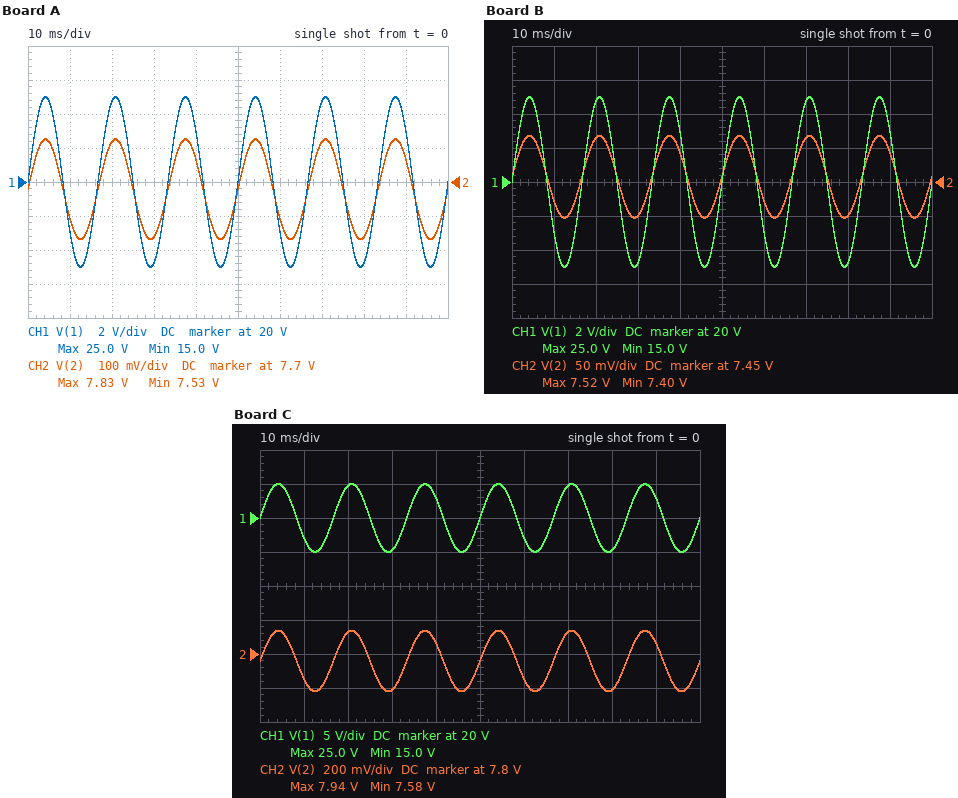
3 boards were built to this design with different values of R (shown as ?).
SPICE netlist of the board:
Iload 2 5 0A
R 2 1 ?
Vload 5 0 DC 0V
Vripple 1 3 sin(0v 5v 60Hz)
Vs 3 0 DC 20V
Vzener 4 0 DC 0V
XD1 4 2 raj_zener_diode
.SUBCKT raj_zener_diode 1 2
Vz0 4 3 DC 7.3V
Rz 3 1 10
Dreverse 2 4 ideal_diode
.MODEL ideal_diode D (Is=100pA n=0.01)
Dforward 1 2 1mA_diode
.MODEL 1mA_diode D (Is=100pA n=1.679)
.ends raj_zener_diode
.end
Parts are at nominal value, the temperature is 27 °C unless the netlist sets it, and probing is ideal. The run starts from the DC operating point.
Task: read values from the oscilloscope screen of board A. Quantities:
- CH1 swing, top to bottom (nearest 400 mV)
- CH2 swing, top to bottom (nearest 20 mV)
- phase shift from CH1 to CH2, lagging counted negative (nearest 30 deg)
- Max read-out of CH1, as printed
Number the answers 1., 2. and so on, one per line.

1. 10.0 V
2. 300 mV
3. 0 deg
4. 25.0 V
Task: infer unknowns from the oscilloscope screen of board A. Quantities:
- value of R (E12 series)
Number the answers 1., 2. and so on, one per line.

1. 330 Ω
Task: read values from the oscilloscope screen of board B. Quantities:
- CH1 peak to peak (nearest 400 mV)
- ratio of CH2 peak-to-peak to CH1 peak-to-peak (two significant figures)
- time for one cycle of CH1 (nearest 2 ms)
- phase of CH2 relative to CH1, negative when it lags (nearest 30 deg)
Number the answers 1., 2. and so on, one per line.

1. 10.0 V
2. 0.012
3. 16 ms
4. 0 deg
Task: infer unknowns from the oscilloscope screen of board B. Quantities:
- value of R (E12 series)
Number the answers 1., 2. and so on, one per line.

1. 820 Ω
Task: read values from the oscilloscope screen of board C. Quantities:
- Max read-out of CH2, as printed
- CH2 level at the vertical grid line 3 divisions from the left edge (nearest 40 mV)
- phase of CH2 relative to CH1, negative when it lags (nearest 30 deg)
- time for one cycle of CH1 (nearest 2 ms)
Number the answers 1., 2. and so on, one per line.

1. 7.94 V
2. 7.60 V
3. 0 deg
4. 16 ms
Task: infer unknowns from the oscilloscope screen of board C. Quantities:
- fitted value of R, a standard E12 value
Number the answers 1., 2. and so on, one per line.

1. 270 Ω
